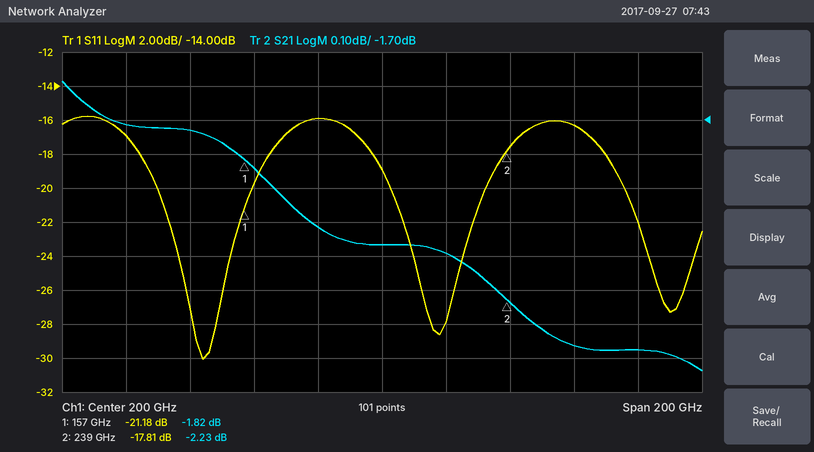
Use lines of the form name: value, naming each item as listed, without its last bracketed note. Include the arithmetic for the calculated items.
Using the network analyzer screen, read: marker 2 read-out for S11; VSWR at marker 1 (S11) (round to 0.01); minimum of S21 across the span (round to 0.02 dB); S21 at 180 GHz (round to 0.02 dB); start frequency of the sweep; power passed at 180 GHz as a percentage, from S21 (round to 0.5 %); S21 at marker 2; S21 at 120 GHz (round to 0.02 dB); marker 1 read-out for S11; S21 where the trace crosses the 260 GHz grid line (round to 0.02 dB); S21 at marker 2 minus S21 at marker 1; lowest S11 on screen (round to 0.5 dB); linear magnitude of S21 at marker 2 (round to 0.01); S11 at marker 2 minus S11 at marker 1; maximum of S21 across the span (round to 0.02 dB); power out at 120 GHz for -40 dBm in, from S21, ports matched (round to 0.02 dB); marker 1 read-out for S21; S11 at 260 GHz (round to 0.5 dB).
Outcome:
marker 2 read-out for S11: -17.81 dB
VSWR at marker 1 (S11): (1 + 0.0873)/(1 − 0.0873) ≈ 1.19
minimum of S21 across the span: -2.44 dB
S21 at 180 GHz: -2.02 dB
start frequency of the sweep: 100 GHz
power passed at 180 GHz as a percentage, from S21: 10^(-2.02/10) ≈ 62.8 %, so 63.0 % to the nearest 0.5 %
S21 at marker 2: -2.23 dB
S21 at 120 GHz: -1.72 dB
marker 1 read-out for S11: -21.18 dB
S21 where the trace crosses the 260 GHz grid line: -2.36 dB
S21 at marker 2 minus S21 at marker 1: -2.23 − (-1.82) = -0.41 dB
lowest S11 on screen: -30.0 dB
linear magnitude of S21 at marker 2: 10^(-2.23/20) ≈ 0.77
S11 at marker 2 minus S11 at marker 1: -17.81 − (-21.18) = 3.37 dB
maximum of S21 across the span: -1.58 dB
power out at 120 GHz for -40 dBm in, from S21, ports matched: -40 dBm + (-1.72 dB) = -41.72 dBm
marker 1 read-out for S21: -1.82 dB
S11 at 260 GHz: -16.5 dB
